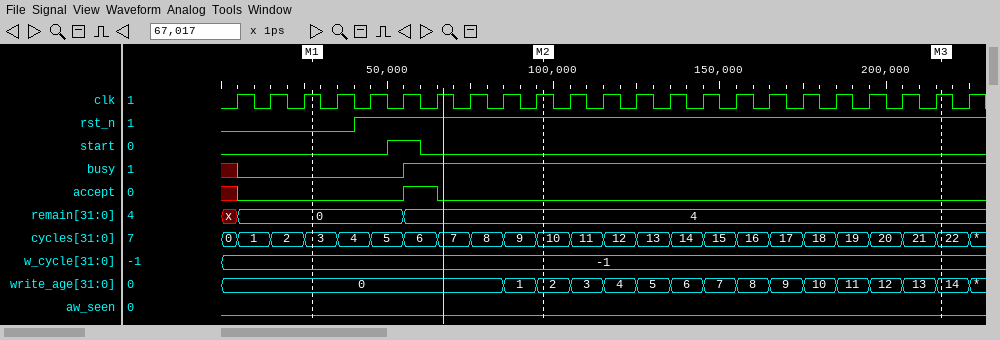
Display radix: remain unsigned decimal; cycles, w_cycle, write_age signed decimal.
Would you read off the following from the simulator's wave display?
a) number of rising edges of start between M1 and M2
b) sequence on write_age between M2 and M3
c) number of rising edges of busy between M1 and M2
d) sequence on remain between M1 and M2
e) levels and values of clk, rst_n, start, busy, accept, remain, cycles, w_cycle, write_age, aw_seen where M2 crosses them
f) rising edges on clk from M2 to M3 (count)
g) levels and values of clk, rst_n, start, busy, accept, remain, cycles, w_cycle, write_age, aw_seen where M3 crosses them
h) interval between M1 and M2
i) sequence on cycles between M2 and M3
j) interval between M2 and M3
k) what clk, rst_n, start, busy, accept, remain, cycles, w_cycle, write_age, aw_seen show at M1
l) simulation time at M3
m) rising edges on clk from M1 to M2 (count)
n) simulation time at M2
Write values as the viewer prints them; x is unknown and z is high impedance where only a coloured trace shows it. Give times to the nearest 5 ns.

1
2, 3, 4, 5, 6, 7, 8, 9, 10, 11, 12, 13, 14
1
0, 4
clk=1, rst_n=1, start=0, busy=1, accept=0, remain=4, cycles=10, w_cycle=-1, write_age=2, aw_seen=0
12
clk=1, rst_n=1, start=0, busy=1, accept=0, remain=4, cycles=22, w_cycle=-1, write_age=14, aw_seen=0
70 ns
10, 11, 12, 13, 14, 15, 16, 17, 18, 19, 20, 21, 22
120 ns
clk=1, rst_n=0, start=0, busy=0, accept=0, remain=0, cycles=3, w_cycle=-1, write_age=0, aw_seen=0
215 ns
7
95 ns
